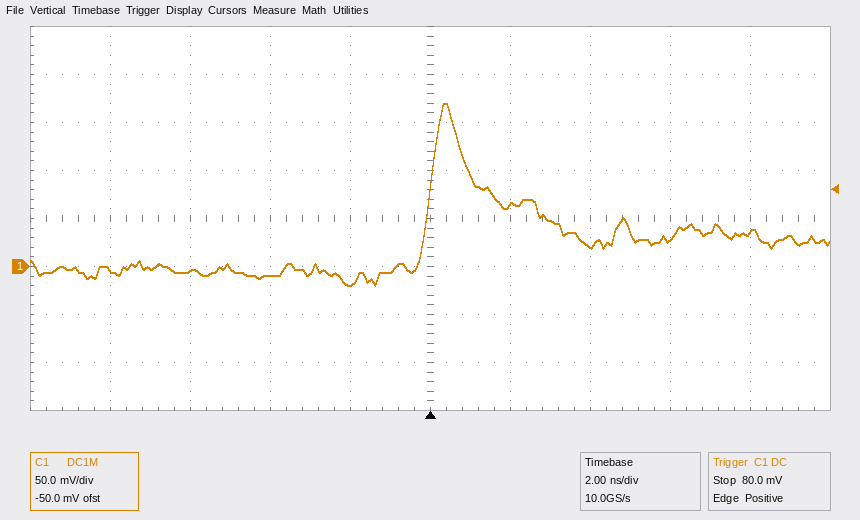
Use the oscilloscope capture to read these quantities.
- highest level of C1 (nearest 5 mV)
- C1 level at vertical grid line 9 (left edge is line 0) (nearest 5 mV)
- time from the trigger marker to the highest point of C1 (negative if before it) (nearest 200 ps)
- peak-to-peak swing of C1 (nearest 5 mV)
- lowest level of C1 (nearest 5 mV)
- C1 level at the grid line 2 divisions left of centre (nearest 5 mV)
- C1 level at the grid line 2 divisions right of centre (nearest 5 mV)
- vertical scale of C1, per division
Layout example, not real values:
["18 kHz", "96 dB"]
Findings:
["170 mV", "35 mV", "+400 ps", "190 mV", "-20 mV", "-10 mV", "20 mV", "50 mV"]
